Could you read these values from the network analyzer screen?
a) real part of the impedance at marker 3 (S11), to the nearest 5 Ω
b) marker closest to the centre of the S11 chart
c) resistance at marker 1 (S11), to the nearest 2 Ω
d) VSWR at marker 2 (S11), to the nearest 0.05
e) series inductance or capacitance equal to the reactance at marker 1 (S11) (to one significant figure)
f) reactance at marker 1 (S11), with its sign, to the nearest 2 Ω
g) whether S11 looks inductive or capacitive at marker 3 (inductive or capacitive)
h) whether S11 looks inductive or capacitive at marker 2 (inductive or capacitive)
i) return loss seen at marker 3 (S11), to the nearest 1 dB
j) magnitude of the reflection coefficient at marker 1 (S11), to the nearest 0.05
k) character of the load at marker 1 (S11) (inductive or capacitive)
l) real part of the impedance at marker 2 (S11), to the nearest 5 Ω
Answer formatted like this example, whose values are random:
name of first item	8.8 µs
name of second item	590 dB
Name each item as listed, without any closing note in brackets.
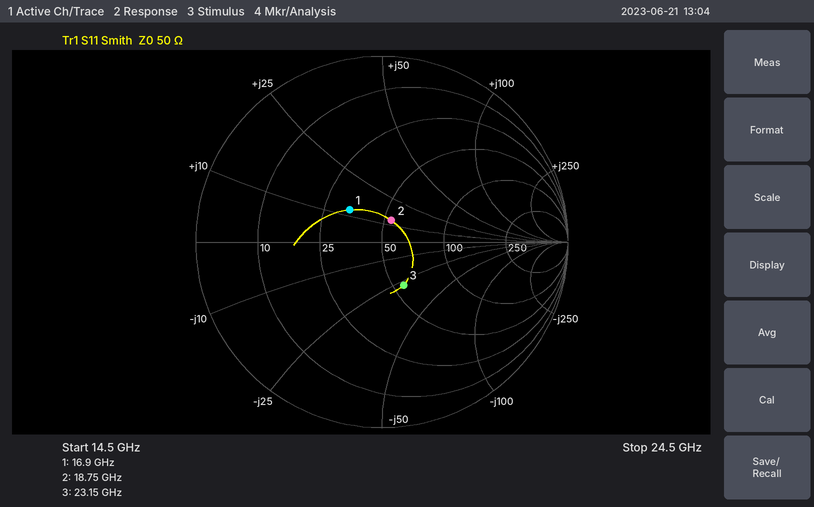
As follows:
real part of the impedance at marker 3 (S11), to the nearest 5 Ω	55 Ω
marker closest to the centre of the S11 chart	marker 2
resistance at marker 1 (S11), to the nearest 2 Ω	34 Ω
VSWR at marker 2 (S11), to the nearest 0.05	1.30
series inductance or capacitance equal to the reactance at marker 1 (S11)	100 pH
reactance at marker 1 (S11), with its sign, to the nearest 2 Ω	+12 Ω
whether S11 looks inductive or capacitive at marker 3	capacitive
whether S11 looks inductive or capacitive at marker 2	inductive
return loss seen at marker 3 (S11), to the nearest 1 dB	12 dB
magnitude of the reflection coefficient at marker 1 (S11), to the nearest 0.05	0.25
character of the load at marker 1 (S11)	inductive
real part of the impedance at marker 2 (S11), to the nearest 5 Ω	55 Ω
